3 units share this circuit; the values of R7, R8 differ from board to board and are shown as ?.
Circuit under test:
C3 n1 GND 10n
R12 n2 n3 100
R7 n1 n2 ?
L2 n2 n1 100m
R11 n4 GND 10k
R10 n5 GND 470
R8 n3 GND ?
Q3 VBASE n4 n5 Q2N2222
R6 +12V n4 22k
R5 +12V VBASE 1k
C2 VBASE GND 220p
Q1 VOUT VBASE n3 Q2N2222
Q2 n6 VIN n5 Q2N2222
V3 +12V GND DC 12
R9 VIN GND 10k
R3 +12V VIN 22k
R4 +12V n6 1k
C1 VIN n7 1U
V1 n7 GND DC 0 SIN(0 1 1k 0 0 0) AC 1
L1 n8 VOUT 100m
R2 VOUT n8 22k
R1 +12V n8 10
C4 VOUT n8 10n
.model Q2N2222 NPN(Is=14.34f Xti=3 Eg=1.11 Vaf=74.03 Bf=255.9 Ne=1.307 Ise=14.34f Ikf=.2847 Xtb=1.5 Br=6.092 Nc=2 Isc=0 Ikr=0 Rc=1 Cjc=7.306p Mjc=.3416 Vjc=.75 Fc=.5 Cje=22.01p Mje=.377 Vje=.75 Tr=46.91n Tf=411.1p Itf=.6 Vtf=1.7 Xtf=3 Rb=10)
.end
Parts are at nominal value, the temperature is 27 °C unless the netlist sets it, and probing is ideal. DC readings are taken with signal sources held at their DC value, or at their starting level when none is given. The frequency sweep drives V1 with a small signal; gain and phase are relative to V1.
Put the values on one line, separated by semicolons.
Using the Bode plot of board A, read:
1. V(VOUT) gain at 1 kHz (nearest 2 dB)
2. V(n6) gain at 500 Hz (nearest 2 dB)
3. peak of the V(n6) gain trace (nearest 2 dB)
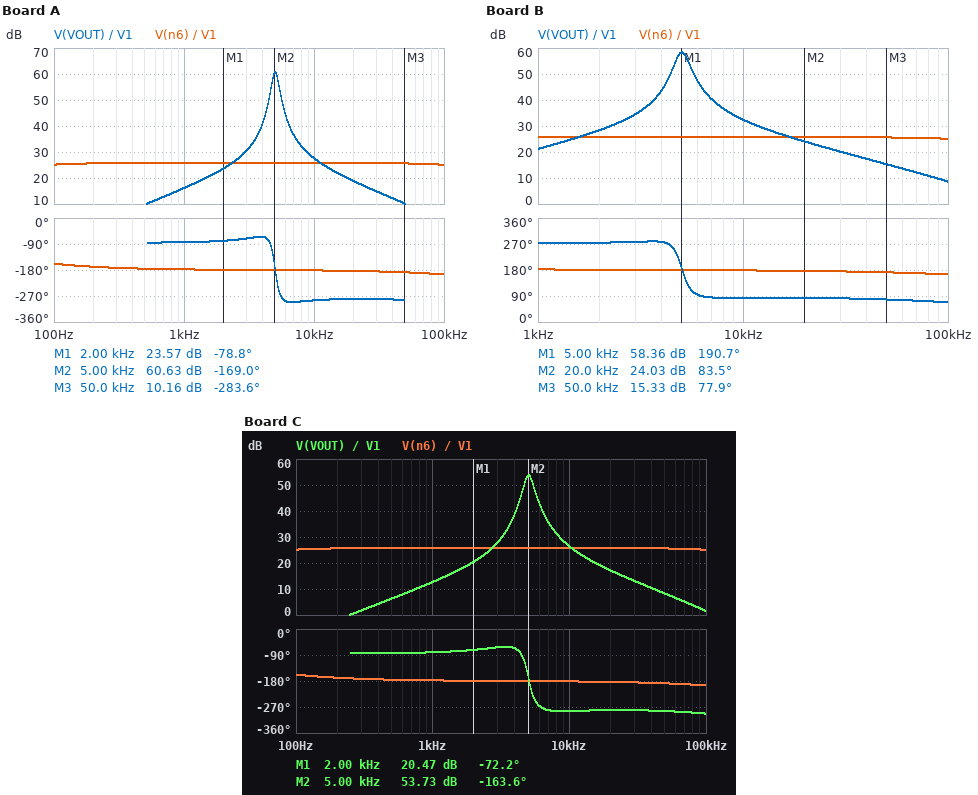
16 dB; 26 dB; 26 dB
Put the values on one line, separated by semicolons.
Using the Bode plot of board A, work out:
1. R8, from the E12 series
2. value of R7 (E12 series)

1.8 kΩ; 33 kΩ
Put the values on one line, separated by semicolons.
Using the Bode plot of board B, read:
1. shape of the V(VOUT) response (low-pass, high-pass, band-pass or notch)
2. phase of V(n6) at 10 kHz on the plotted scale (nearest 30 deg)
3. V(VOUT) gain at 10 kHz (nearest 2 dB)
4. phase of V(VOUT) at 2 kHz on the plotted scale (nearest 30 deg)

band-pass; 180 deg; 32 dB; 270 deg
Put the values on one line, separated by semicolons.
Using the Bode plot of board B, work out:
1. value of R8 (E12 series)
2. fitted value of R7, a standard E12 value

1 kΩ; 15 kΩ
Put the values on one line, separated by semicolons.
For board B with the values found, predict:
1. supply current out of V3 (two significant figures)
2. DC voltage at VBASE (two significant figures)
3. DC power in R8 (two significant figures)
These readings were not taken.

15 mA; 8.8 V; 66 mW
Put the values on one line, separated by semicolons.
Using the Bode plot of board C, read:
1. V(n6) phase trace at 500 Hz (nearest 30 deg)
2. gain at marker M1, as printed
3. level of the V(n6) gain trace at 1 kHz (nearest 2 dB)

-180 deg; 20.47 dB; 26 dB
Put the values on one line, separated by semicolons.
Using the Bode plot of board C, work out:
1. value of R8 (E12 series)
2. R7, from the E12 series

2.7 kΩ; 10 kΩ
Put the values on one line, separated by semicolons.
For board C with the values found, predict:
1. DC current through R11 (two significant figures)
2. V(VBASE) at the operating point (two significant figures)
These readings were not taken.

360 µA; 8.9 V
